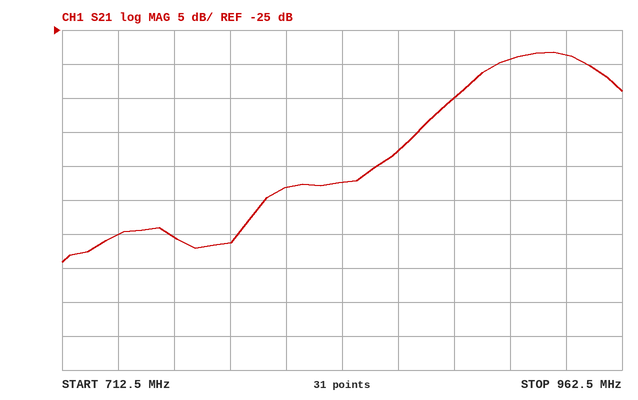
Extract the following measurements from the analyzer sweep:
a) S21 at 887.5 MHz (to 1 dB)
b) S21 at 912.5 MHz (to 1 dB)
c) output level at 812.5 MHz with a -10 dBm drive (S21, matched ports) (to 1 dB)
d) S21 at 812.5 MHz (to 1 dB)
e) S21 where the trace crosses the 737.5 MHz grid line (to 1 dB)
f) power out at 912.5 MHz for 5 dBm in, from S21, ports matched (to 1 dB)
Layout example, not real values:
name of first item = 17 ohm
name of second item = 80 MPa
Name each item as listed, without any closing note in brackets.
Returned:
S21 at 887.5 MHz = -35 dB
S21 at 912.5 MHz = -29 dB
output level at 812.5 MHz with a -10 dBm drive (S21, matched ports) = -58 dBm
S21 at 812.5 MHz = -48 dB
S21 where the trace crosses the 737.5 MHz grid line = -55 dB
power out at 912.5 MHz for 5 dBm in, from S21, ports matched = -24 dBm
